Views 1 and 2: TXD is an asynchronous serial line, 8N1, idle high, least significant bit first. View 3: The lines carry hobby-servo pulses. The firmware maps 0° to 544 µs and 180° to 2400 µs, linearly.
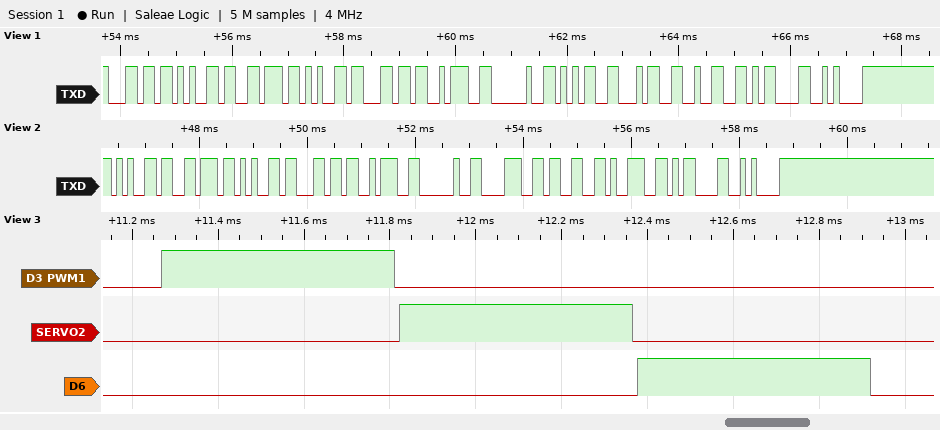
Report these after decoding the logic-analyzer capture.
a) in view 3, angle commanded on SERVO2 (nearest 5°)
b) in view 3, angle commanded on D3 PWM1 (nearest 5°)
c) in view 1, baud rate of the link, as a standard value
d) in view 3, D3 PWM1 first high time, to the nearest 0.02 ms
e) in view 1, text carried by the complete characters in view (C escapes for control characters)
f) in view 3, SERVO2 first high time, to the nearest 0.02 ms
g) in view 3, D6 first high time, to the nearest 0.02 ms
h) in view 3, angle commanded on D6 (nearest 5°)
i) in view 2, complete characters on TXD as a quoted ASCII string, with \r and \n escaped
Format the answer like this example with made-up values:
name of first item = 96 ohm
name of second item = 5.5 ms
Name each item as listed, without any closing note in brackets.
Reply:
in view 3, angle commanded on SERVO2 = 0°
in view 3, angle commanded on D3 PWM1 = 0°
in view 1, baud rate of the link, as a standard value = 9600 baud
in view 3, D3 PWM1 first high time, to the nearest 0.02 ms = 0.54 ms
in view 1, text carried by the complete characters in view = "level: 542\r\n"
in view 3, SERVO2 first high time, to the nearest 0.02 ms = 0.54 ms
in view 3, D6 first high time, to the nearest 0.02 ms = 0.54 ms
in view 3, angle commanded on D6 = 0°
in view 2, complete characters on TXD as a quoted ASCII string, with \r and \n escaped = "evel: 839\r\n"
